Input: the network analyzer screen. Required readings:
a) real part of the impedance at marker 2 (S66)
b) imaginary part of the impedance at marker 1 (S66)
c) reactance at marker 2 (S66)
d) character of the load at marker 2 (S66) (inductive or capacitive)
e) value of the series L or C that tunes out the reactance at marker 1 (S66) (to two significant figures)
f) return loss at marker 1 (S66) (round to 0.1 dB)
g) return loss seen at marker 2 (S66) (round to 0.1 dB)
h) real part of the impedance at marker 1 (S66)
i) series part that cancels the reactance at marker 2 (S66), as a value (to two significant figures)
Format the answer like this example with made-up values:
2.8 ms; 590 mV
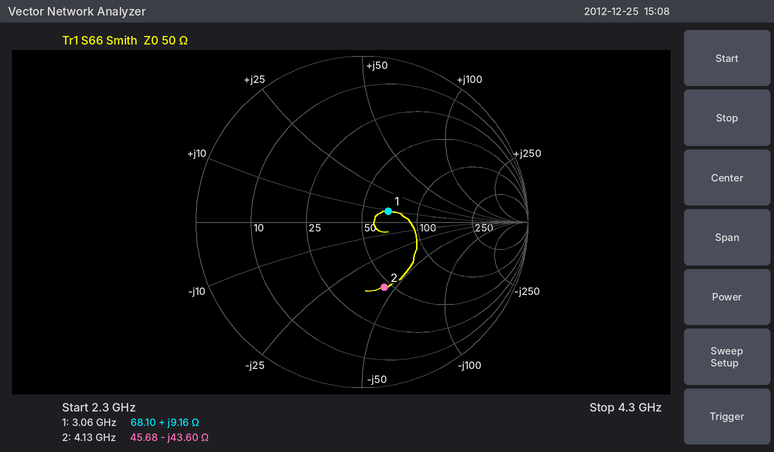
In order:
45.68 Ω; +9.16 Ω; -43.60 Ω; capacitive; 5.7 pF; 15.3 dB; 7.6 dB; 68.10 Ω; 1.7 nH
